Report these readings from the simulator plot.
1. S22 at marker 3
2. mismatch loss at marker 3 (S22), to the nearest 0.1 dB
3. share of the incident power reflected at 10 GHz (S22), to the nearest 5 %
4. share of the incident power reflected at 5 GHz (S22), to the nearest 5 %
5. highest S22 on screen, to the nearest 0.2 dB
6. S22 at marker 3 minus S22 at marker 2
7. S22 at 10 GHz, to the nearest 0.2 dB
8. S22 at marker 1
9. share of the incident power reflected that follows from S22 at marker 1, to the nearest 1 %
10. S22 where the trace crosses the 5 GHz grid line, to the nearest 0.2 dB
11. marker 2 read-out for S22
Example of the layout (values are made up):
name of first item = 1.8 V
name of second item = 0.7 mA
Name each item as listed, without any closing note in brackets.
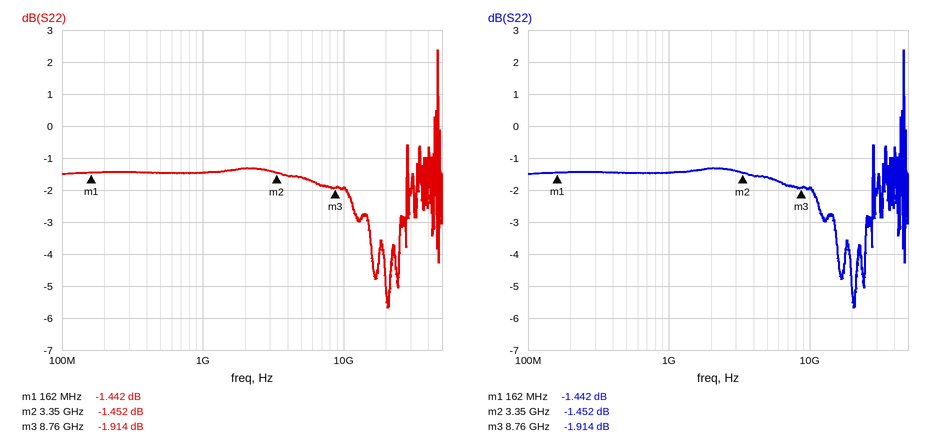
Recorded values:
S22 at marker 3 = -1.914 dB
mismatch loss at marker 3 (S22), to the nearest 0.1 dB = 4.5 dB
share of the incident power reflected at 10 GHz (S22), to the nearest 5 % = 65 %
share of the incident power reflected at 5 GHz (S22), to the nearest 5 % = 70 %
highest S22 on screen, to the nearest 0.2 dB = 2.4 dB
S22 at marker 3 minus S22 at marker 2 = -0.462 dB
S22 at 10 GHz, to the nearest 0.2 dB = -2.0 dB
S22 at marker 1 = -1.442 dB
share of the incident power reflected that follows from S22 at marker 1, to the nearest 1 % = 72 %
S22 where the trace crosses the 5 GHz grid line, to the nearest 0.2 dB = -1.6 dB
marker 2 read-out for S22 = -1.452 dB
